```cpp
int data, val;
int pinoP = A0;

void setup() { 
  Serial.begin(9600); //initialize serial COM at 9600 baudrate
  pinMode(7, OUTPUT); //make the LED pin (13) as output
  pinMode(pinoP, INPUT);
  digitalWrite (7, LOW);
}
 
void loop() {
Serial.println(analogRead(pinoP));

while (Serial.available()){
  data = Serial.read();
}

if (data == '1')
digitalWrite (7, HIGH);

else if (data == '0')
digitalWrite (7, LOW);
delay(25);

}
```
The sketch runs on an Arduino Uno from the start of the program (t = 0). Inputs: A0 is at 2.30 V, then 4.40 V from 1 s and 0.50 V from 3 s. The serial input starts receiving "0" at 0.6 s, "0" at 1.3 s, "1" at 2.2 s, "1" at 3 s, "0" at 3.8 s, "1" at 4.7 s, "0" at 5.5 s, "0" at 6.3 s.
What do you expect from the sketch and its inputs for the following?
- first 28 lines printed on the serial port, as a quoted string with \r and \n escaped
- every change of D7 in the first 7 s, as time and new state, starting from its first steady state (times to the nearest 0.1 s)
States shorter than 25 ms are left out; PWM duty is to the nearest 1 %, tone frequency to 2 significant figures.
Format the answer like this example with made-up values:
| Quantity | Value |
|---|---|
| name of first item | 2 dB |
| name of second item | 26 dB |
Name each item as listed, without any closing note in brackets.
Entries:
| Quantity | Value |
|---|---|
| first 28 lines printed on the serial port, as a quoted string with \r and \n escaped | "471\r\n471\r\n471\r\n471\r\n471\r\n471\r\n471\r\n471\r\n471\r\n471\r\n471\r\n471\r\n471\r\n471\r\n471\r\n471\r\n471\r\n471\r\n471\r\n471\r\n471\r\n471\r\n471\r\n471\r\n471\r\n471\r\n471\r\n471\r\n" |
| every change of D7 in the first 7 s, as time and new state, starting from its first steady state | 0 s low; 2.2 s high; 3.8 s low; 4.7 s high; 5.5 s low |
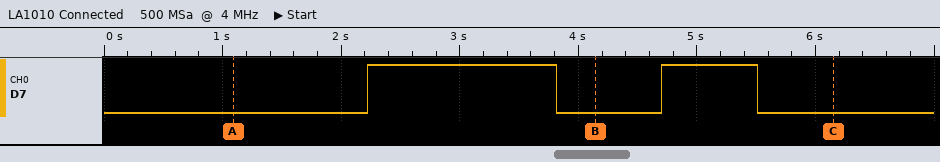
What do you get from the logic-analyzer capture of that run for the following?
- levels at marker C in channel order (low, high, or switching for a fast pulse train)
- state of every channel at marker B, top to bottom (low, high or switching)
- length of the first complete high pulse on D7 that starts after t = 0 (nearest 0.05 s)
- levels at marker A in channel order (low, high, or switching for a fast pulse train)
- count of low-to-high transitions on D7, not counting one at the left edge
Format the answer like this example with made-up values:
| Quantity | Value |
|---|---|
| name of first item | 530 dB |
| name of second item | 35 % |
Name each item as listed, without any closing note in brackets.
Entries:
| Quantity | Value |
|---|---|
| levels at marker C in channel order | D7 low |
| state of every channel at marker B, top to bottom | D7 low |
| length of the first complete high pulse on D7 that starts after t = 0 | 1.60 s |
| levels at marker A in channel order | D7 low |
| count of low-to-high transitions on D7, not counting one at the left edge | 2 |
